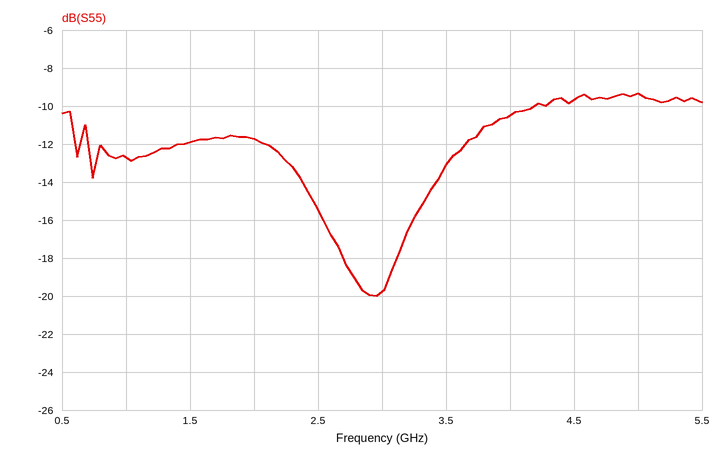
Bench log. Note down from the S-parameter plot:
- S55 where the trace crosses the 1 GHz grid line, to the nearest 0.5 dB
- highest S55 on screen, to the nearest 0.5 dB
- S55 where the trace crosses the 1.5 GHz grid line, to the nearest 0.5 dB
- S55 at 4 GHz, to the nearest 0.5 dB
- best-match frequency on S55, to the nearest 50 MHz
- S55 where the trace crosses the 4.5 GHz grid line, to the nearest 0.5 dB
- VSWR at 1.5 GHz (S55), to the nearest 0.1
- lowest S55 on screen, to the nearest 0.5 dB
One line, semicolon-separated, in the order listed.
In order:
-12.5 dB; -9.5 dB; -12.0 dB; -10.5 dB; 2.95 GHz; -9.5 dB; 1.7; -20.0 dB
